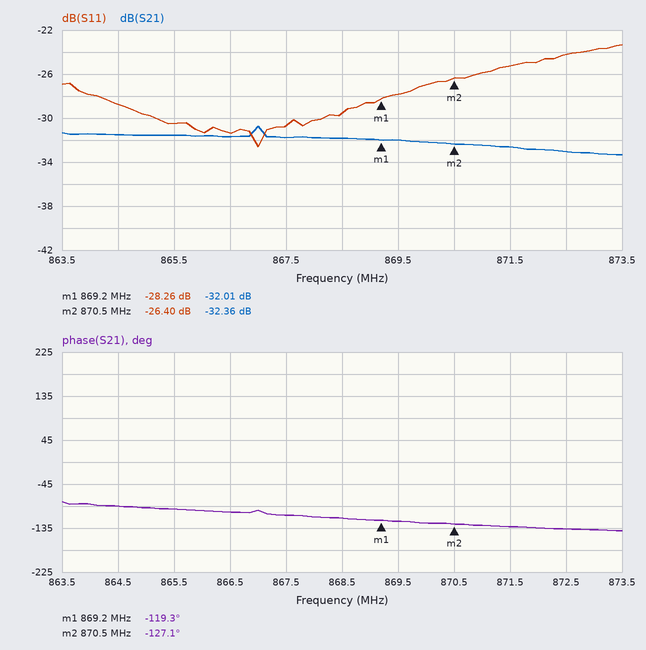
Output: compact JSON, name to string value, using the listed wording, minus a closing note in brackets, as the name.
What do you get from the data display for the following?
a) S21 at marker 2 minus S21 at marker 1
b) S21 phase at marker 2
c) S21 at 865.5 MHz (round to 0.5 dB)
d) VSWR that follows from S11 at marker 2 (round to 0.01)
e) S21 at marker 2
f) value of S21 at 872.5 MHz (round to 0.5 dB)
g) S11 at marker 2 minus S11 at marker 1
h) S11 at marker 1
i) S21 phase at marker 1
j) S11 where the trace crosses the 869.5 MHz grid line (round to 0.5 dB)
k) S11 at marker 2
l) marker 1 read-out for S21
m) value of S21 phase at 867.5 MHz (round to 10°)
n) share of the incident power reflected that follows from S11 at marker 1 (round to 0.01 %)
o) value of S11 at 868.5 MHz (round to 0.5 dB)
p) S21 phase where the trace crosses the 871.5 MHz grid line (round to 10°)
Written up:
{"S21 at marker 2 minus S21 at marker 1": "-0.35 dB", "S21 phase at marker 2": "-127.1°", "S21 at 865.5 MHz": "-31.5 dB", "VSWR that follows from S11 at marker 2": "1.10", "S21 at marker 2": "-32.36 dB", "value of S21 at 872.5 MHz": "-33.0 dB", "S11 at marker 2 minus S11 at marker 1": "1.86 dB", "S11 at marker 1": "-28.26 dB", "S21 phase at marker 1": "-119.3°", "S11 where the trace crosses the 869.5 MHz grid line": "-28.0 dB", "S11 at marker 2": "-26.40 dB", "marker 1 read-out for S21": "-32.01 dB", "value of S21 phase at 867.5 MHz": "-110°", "share of the incident power reflected that follows from S11 at marker 1": "0.15 %", "value of S11 at 868.5 MHz": "-29.5 dB", "S21 phase where the trace crosses the 871.5 MHz grid line": "-130°"}
